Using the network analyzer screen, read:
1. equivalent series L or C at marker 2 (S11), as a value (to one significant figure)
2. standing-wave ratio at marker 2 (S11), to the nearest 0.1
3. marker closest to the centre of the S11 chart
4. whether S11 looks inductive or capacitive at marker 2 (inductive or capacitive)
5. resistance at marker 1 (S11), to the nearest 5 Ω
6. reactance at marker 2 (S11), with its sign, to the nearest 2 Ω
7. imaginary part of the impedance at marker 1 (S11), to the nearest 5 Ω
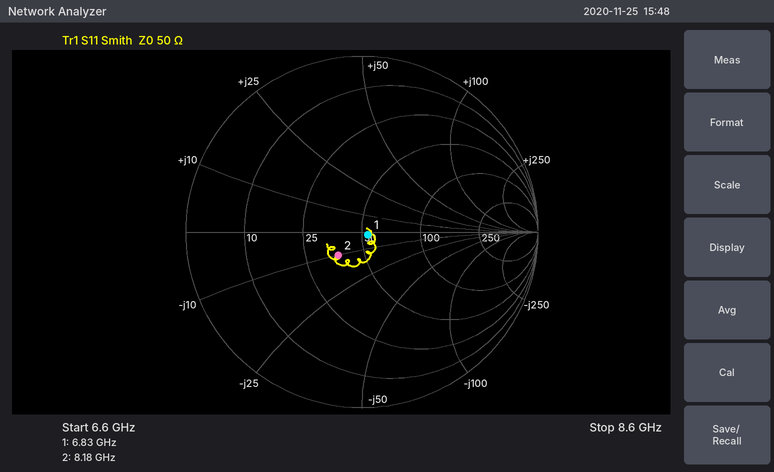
2 pF
1.5
marker 1
capacitive
55 Ω
-10 Ω
0 Ω
